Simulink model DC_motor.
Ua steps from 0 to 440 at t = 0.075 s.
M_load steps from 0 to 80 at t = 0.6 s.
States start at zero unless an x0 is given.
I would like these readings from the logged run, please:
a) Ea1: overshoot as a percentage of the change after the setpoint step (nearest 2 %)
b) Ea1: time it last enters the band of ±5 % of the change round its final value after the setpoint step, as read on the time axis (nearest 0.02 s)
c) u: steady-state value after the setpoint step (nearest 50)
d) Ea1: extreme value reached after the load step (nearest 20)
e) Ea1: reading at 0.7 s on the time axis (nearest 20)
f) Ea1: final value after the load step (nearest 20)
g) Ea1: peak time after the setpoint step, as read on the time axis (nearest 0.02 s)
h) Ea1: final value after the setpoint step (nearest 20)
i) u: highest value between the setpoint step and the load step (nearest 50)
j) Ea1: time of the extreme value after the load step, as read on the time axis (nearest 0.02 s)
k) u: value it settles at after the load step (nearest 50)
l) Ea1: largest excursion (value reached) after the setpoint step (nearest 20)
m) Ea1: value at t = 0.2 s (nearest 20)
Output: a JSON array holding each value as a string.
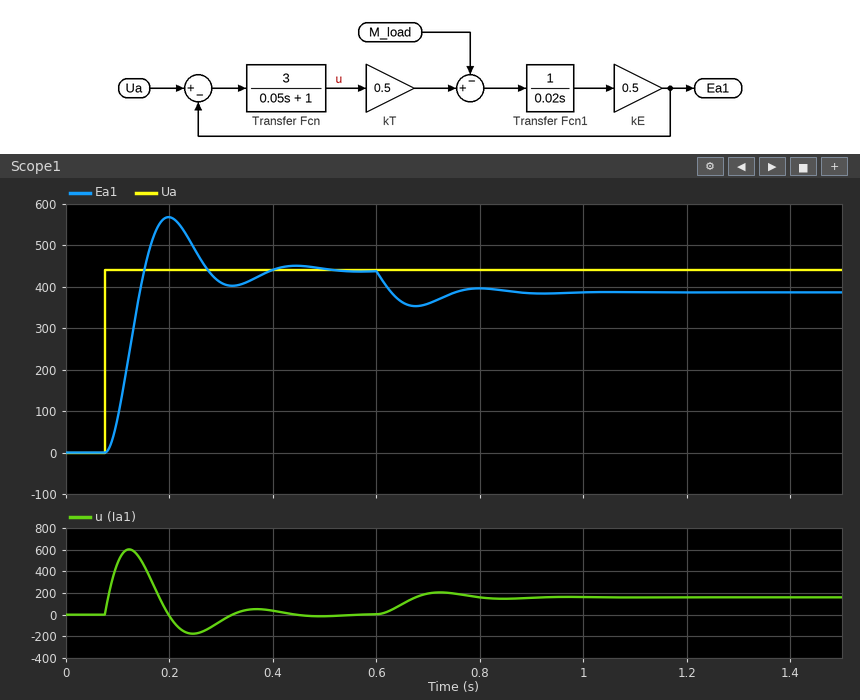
["30 %", "0.36 s", "0", "360", "360", "380", "0.20 s", "440", "600", "0.68 s", "150", "560", "560"]
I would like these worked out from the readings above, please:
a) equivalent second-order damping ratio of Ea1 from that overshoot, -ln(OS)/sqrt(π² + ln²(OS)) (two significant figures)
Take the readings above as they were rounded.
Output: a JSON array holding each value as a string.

["0.36"]
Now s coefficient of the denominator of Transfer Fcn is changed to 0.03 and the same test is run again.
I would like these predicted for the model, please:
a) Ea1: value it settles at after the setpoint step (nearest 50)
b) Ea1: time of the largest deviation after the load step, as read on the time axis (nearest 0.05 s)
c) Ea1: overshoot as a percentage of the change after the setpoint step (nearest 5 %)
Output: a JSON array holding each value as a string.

["450", "0.65 s", "20 %"]
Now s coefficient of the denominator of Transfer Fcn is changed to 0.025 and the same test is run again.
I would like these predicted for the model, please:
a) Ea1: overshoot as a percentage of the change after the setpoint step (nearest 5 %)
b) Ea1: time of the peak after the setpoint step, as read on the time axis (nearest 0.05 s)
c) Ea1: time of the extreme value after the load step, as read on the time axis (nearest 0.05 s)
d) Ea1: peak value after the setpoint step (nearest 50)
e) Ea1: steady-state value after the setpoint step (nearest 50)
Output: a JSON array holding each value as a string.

["15 %", "0.15 s", "0.65 s", "500", "450"]
